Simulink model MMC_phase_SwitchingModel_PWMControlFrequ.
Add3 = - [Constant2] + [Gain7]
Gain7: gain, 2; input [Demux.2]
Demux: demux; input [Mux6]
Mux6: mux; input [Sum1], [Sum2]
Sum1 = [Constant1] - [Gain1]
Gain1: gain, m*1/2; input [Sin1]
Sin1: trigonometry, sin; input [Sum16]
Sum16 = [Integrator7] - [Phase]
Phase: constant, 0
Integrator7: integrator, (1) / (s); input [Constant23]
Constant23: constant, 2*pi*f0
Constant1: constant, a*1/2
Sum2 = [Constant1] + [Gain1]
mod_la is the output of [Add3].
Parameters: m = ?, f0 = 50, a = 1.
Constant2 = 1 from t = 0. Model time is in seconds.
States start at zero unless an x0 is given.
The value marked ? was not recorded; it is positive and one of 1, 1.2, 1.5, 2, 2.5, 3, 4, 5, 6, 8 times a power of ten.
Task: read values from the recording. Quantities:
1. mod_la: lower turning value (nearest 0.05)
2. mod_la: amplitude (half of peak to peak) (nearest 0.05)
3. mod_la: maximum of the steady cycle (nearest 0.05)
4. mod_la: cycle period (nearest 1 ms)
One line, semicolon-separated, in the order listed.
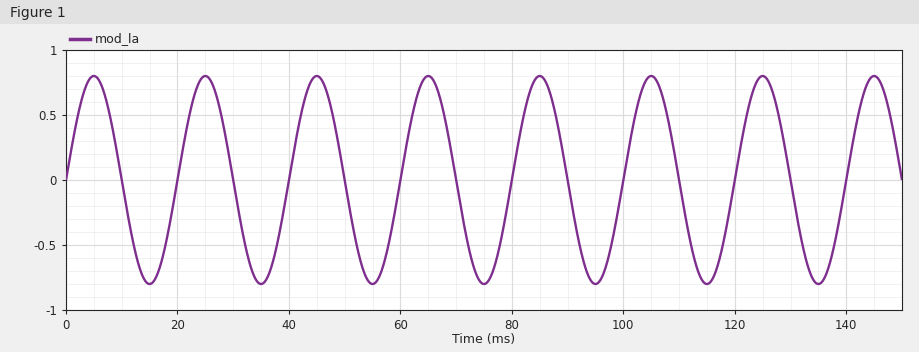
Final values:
-0.80; 0.80; 0.80; 20 ms
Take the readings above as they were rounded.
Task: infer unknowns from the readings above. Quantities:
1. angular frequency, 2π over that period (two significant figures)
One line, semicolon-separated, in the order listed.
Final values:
0.31 rad/ms
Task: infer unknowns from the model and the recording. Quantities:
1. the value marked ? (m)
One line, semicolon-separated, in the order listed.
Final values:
0.8
